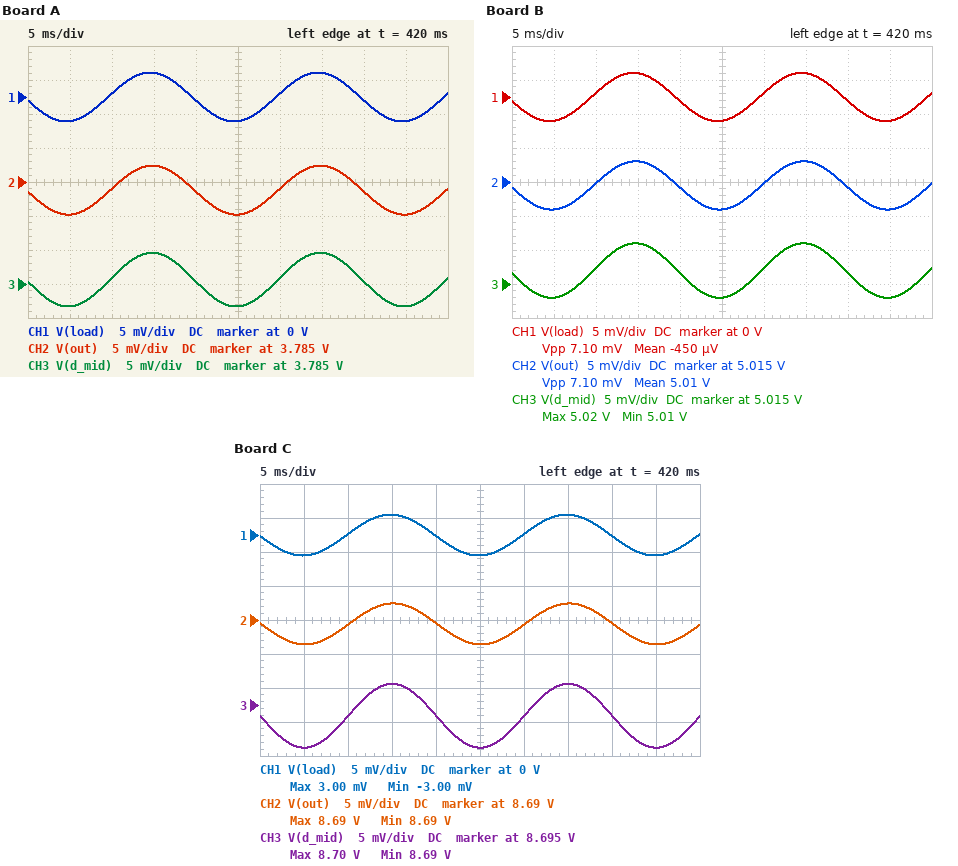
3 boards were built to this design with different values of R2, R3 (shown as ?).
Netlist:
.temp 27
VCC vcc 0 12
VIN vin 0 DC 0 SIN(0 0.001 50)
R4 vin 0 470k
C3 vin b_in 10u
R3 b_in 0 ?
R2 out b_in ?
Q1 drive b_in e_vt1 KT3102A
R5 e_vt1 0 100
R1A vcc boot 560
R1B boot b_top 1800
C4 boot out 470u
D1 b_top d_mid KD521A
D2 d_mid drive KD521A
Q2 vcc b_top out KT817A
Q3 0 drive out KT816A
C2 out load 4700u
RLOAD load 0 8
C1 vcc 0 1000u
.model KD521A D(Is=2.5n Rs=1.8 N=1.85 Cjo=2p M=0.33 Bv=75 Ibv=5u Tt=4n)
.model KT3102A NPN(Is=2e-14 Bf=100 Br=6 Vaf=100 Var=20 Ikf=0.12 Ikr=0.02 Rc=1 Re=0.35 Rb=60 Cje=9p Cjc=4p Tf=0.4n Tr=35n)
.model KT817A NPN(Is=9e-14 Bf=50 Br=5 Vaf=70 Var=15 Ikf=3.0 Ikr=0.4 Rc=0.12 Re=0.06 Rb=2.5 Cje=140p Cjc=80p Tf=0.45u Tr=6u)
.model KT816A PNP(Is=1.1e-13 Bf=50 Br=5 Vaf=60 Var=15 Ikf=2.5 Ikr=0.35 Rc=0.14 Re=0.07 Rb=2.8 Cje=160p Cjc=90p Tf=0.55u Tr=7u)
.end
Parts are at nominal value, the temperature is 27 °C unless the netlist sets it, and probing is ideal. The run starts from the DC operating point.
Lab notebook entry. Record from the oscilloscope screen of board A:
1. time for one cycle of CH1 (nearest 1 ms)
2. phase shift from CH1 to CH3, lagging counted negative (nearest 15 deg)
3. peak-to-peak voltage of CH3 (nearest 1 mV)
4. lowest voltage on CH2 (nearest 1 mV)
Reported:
20 ms
0 deg
8 mV
3.780 V
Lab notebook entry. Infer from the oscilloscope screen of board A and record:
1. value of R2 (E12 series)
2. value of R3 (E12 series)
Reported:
18 kΩ
8.2 kΩ
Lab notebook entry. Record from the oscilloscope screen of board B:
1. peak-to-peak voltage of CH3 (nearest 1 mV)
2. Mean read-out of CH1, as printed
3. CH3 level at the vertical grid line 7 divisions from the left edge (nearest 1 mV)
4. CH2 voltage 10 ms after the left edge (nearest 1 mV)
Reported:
8 mV
-450 µV
5.021 V
5.015 V
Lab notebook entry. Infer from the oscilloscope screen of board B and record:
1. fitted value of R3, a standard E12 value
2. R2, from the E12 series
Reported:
4.7 kΩ
18 kΩ
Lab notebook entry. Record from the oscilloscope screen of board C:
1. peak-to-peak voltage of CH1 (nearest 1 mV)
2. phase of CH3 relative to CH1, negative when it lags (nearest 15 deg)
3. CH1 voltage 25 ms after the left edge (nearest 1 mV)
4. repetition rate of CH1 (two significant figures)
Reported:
6 mV
0 deg
-3 mV
50 Hz
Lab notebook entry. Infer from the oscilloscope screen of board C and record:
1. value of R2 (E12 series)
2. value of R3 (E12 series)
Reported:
150 kΩ
18 kΩ
